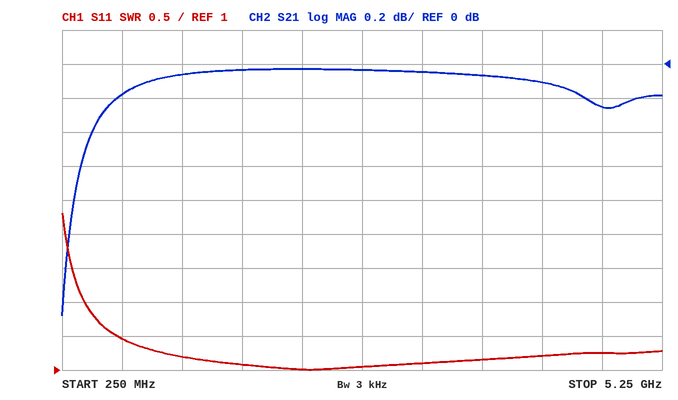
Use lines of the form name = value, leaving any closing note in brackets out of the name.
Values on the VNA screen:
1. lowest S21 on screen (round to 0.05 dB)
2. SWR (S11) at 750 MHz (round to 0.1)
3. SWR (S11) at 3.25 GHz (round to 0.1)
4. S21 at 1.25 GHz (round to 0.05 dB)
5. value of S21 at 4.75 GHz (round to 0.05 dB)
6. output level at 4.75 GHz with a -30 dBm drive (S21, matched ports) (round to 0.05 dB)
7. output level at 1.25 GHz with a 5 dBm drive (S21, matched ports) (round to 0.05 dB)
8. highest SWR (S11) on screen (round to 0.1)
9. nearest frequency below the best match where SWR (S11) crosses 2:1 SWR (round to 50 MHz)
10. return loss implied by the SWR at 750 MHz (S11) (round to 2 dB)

lowest S21 on screen = -1.50 dB
SWR (S11) at 750 MHz = 1.5
SWR (S11) at 3.25 GHz = 1.1
S21 at 1.25 GHz = -0.05 dB
value of S21 at 4.75 GHz = -0.25 dB
output level at 4.75 GHz with a -30 dBm drive (S21, matched ports) = -30.25 dBm
output level at 1.25 GHz with a 5 dBm drive (S21, matched ports) = 4.95 dBm
highest SWR (S11) on screen = 3.3
nearest frequency below the best match where SWR (S11) crosses 2:1 SWR = 450 MHz
return loss implied by the SWR at 750 MHz (S11) = 14 dB
